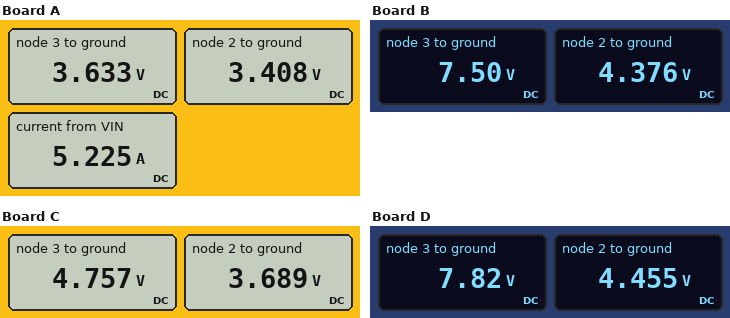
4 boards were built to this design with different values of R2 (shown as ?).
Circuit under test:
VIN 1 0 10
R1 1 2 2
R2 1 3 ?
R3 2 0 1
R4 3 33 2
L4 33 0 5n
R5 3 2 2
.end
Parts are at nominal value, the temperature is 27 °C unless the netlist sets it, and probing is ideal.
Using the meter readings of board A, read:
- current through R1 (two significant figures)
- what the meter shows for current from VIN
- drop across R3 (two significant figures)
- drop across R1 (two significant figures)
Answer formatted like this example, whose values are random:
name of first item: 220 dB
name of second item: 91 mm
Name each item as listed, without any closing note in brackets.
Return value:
current through R1: 3.3 A
what the meter shows for current from VIN: 5.225 A
drop across R3: 3.4 V
drop across R1: 6.6 V
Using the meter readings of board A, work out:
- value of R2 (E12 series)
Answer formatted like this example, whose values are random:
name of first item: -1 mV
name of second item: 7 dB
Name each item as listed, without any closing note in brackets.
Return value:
value of R2: 3.3 Ω
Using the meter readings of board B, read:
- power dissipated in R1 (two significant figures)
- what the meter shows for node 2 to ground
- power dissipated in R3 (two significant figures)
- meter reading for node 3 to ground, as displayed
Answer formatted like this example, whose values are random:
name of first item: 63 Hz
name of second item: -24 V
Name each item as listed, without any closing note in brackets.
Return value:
power dissipated in R1: 16 W
what the meter shows for node 2 to ground: 4.376 V
power dissipated in R3: 19 W
meter reading for node 3 to ground, as displayed: 7.50 V
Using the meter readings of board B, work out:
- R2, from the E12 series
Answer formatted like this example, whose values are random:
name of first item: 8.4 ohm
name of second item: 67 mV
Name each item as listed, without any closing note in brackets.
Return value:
R2, from the E12 series: 0.47 Ω
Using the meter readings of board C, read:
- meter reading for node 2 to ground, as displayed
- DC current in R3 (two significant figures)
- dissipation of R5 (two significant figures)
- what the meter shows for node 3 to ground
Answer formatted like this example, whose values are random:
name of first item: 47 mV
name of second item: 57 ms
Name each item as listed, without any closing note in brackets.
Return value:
meter reading for node 2 to ground, as displayed: 3.689 V
DC current in R3: 3.7 A
dissipation of R5: 570 mW
what the meter shows for node 3 to ground: 4.757 V
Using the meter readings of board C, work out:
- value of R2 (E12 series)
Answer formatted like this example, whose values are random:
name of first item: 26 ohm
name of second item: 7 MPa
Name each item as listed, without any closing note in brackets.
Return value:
value of R2: 1.8 Ω
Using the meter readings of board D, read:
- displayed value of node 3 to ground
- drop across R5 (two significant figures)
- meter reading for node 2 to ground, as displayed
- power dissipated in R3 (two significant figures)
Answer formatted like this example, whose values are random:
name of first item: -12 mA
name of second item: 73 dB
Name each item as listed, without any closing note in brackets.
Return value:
displayed value of node 3 to ground: 7.82 V
drop across R5: 3.4 V
meter reading for node 2 to ground, as displayed: 4.455 V
power dissipated in R3: 20 W
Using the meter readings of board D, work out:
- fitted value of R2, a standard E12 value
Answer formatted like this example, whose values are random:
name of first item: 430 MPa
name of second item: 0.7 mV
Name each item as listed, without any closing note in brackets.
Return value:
fitted value of R2, a standard E12 value: 0.39 Ω
